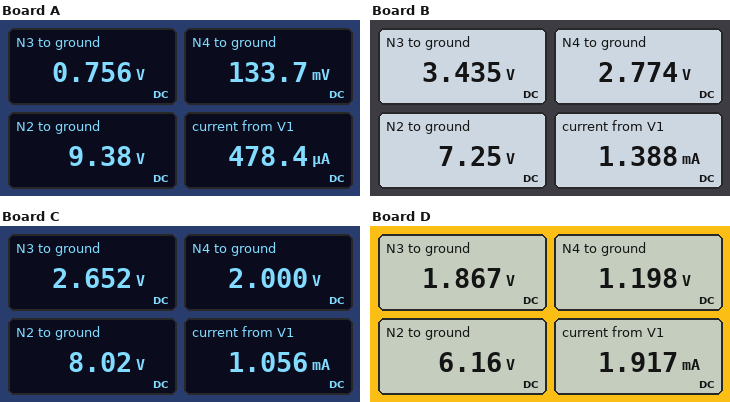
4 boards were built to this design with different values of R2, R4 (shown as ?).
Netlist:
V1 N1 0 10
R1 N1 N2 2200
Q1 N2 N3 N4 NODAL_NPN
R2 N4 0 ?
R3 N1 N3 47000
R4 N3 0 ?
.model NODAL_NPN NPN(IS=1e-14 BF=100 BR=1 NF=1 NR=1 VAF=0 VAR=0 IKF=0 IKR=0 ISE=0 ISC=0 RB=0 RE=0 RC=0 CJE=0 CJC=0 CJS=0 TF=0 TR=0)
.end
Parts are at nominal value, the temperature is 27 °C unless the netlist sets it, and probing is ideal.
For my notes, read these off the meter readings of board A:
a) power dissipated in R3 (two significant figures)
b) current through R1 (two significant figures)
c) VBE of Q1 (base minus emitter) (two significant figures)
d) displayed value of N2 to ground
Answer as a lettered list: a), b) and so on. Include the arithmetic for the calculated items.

a) (10 V - 756 mV)^2 / 47 kΩ = 1.8 mW
b) (10 V - 9.38 V) / 2.2 kΩ = 280 µA
c) 756 mV - 133.7 mV = 620 mV
d) 9.38 V
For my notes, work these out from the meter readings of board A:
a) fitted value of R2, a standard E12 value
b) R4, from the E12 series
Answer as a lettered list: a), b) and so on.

a) 470 Ω
b) 3.9 kΩ
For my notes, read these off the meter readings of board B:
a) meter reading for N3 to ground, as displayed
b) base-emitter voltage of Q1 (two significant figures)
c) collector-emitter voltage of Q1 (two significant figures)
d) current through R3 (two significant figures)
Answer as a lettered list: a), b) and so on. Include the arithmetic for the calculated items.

a) 3.435 V
b) 3.435 V - 2.774 V = 660 mV
c) 7.25 V - 2.774 V = 4.5 V
d) (10 V - 3.435 V) / 47 kΩ = 140 µA
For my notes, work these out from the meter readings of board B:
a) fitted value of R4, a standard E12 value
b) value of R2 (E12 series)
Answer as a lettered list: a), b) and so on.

a) 27 kΩ
b) 2.2 kΩ
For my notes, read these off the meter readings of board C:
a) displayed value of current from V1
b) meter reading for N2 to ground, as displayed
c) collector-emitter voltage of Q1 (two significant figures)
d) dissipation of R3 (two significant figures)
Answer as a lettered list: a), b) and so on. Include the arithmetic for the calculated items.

a) 1.056 mA
b) 8.02 V
c) 8.02 V - 2 V = 6.0 V
d) (10 V - 2.652 V)^2 / 47 kΩ = 1.1 mW
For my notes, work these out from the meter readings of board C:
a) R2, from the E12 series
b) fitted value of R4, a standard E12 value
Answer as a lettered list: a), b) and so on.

a) 2.2 kΩ
b) 18 kΩ
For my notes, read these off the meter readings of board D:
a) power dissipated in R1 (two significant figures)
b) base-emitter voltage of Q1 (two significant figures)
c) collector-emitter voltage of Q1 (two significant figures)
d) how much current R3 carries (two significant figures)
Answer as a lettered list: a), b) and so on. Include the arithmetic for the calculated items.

a) (10 V - 6.16 V)^2 / 2.2 kΩ = 6.7 mW
b) 1.867 V - 1.198 V = 670 mV
c) 6.16 V - 1.198 V = 5.0 V
d) (10 V - 1.867 V) / 47 kΩ = 170 µA
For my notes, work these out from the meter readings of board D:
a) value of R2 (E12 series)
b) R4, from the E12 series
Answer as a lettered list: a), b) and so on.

a) 680 Ω
b) 12 kΩ
